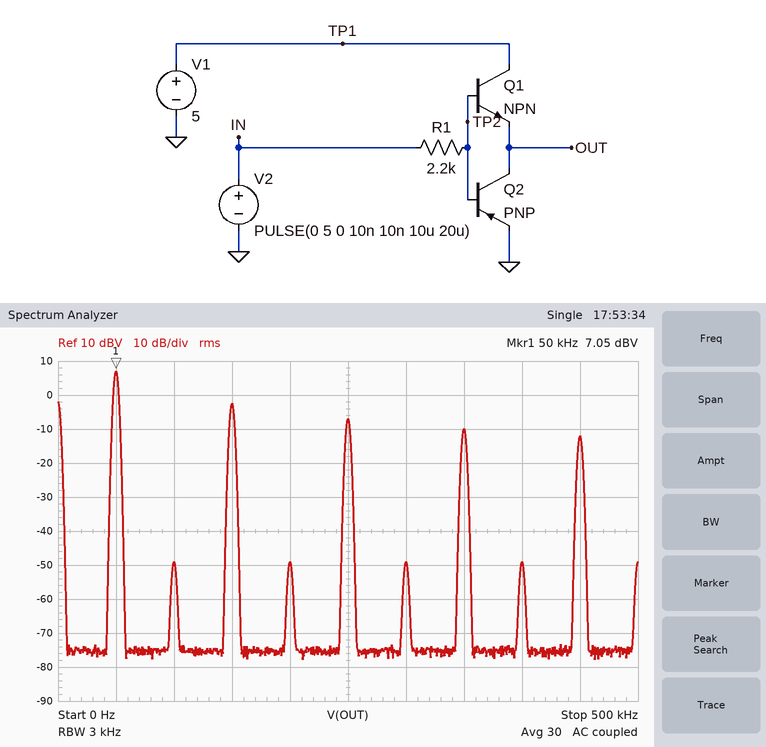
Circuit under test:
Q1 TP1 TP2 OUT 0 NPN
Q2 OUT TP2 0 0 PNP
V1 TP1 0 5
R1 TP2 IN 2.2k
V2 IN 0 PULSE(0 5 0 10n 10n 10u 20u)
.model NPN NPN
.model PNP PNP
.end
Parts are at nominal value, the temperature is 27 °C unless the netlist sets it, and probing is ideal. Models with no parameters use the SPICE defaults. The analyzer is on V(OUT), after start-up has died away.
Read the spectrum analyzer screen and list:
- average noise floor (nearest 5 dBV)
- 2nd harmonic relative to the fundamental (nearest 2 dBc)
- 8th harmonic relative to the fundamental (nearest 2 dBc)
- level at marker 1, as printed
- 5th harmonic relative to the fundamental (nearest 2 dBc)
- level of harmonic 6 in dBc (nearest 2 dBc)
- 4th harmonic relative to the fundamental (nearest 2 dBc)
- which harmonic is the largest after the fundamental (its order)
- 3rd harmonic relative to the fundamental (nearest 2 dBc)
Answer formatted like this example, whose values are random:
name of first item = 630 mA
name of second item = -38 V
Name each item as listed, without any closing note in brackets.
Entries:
average noise floor = -75 dBV
2nd harmonic relative to the fundamental = -56 dBc
8th harmonic relative to the fundamental = -56 dBc
level at marker 1, as printed = 7.05 dBV
5th harmonic relative to the fundamental = -14 dBc
level of harmonic 6 in dBc = -56 dBc
4th harmonic relative to the fundamental = -56 dBc
which harmonic is the largest after the fundamental = 3
3rd harmonic relative to the fundamental = -10 dBc
